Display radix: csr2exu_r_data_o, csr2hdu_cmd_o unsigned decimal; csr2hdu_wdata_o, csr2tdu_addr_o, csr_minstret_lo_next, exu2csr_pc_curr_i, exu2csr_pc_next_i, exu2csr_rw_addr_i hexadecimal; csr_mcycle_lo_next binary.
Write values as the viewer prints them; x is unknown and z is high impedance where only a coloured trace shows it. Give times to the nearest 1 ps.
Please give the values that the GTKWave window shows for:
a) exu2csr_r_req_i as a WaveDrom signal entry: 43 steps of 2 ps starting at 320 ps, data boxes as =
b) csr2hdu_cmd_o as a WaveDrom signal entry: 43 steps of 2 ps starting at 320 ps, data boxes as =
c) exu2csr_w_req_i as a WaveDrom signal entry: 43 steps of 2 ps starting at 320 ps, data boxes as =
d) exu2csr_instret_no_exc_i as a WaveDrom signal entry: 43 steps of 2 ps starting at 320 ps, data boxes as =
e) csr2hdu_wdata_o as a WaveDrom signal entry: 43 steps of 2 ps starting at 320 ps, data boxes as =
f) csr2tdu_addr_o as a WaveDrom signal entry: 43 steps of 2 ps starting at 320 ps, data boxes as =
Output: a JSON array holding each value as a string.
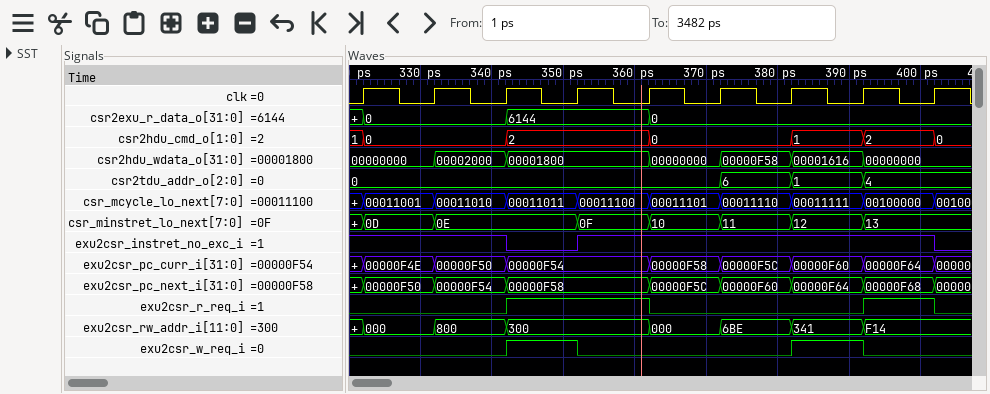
["{name: 'exu2csr_r_req_i', wave: '0..........1.........0..............1....0.'}", "{name: 'csr2hdu_cmd_o', wave: '==.........=.........=.........=....=....=.', data: '1 0 2 0 1 2 0'}", "{name: 'exu2csr_w_req_i', wave: '0..........1....0..............1....0......'}", "{name: 'exu2csr_instret_no_exc_i', wave: '1..........0....1........................0.'}", "{name: 'csr2hdu_wdata_o', wave: '=.....=....=.........=....=....=....=......', data: '00000000 00002000 00001800 00000000 00000F58 00001616 00000000'}", "{name: 'csr2tdu_addr_o', wave: '=.........................=....=....=......', data: '0 6 1 4'}"]
